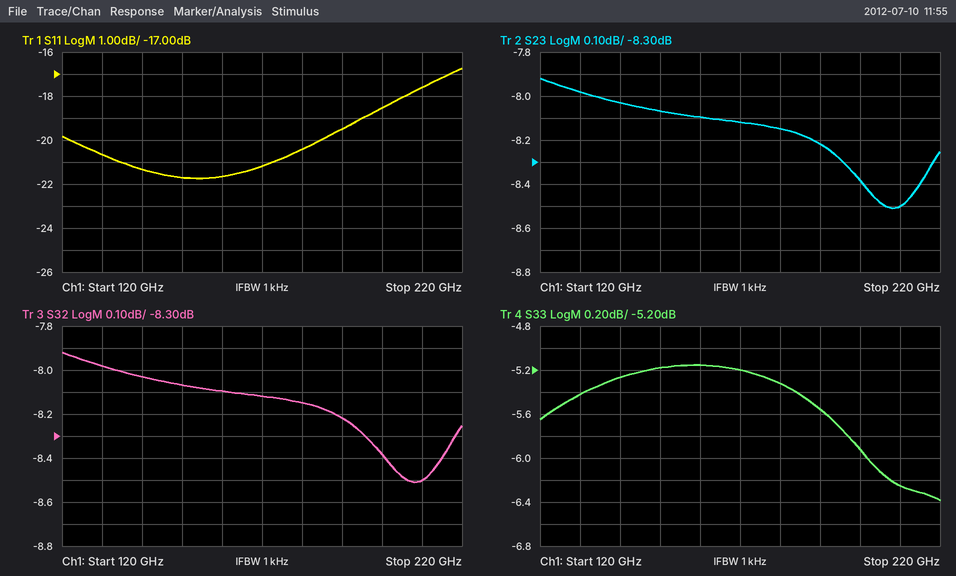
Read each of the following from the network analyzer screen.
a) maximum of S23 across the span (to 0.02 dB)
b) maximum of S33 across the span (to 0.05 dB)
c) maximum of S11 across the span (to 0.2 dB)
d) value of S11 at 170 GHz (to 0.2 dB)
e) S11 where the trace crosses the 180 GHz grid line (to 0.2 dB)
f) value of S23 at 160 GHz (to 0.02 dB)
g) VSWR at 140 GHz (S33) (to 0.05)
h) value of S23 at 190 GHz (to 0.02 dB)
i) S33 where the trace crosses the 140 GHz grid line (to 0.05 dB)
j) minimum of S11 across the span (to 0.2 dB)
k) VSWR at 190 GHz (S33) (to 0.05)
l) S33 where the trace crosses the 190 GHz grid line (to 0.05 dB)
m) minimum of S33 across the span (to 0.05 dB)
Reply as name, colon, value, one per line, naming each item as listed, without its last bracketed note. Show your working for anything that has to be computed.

maximum of S23 across the span: -7.92 dB
maximum of S33 across the span: -5.15 dB
maximum of S11 across the span: -16.8 dB
value of S11 at 170 GHz: -21.2 dB
S11 where the trace crosses the 180 GHz grid line: -20.4 dB
value of S23 at 160 GHz: -8.10 dB
VSWR at 140 GHz (S33): |Γ| = 10^(-5.25/20) = 0.5464; VSWR = (1 + 0.5464)/(1 − 0.5464) ≈ 3.41, so 3.40 to the nearest 0.05
value of S23 at 190 GHz: -8.22 dB
S33 where the trace crosses the 140 GHz grid line: -5.25 dB
minimum of S11 across the span: -21.8 dB
VSWR at 190 GHz (S33): |Γ| = 10^(-5.55/20) = 0.5278; VSWR = (1 + 0.5278)/(1 − 0.5278) ≈ 3.24, so 3.25 to the nearest 0.05
S33 where the trace crosses the 190 GHz grid line: -5.55 dB
minimum of S33 across the span: -6.40 dB
